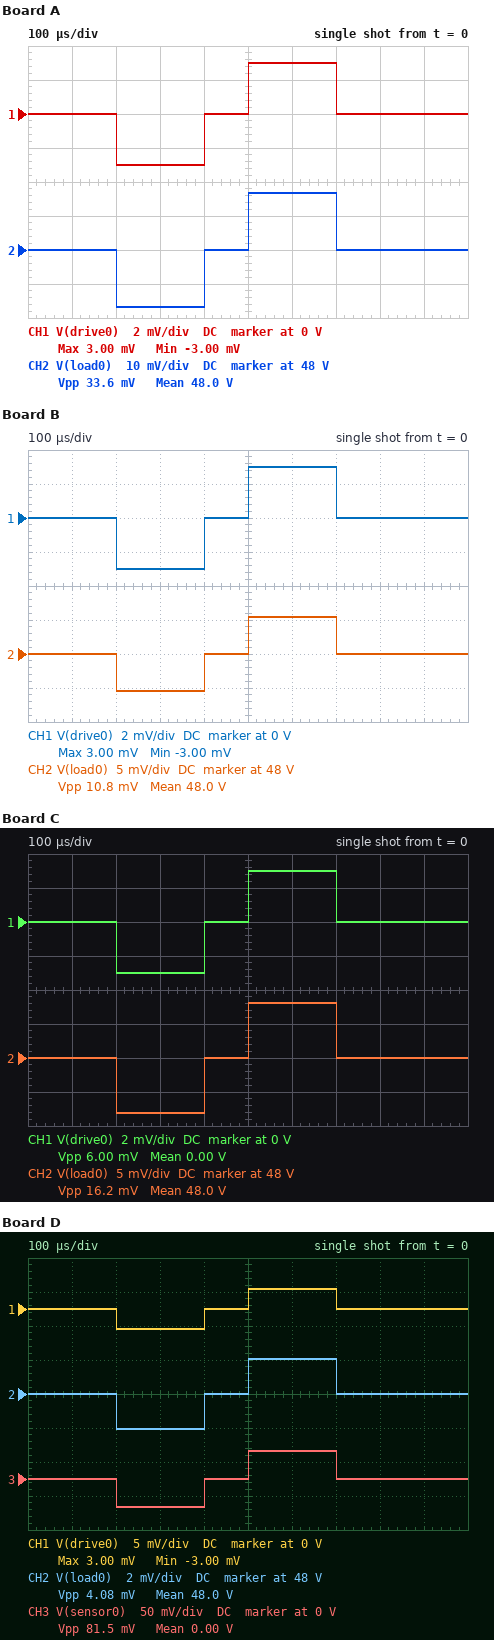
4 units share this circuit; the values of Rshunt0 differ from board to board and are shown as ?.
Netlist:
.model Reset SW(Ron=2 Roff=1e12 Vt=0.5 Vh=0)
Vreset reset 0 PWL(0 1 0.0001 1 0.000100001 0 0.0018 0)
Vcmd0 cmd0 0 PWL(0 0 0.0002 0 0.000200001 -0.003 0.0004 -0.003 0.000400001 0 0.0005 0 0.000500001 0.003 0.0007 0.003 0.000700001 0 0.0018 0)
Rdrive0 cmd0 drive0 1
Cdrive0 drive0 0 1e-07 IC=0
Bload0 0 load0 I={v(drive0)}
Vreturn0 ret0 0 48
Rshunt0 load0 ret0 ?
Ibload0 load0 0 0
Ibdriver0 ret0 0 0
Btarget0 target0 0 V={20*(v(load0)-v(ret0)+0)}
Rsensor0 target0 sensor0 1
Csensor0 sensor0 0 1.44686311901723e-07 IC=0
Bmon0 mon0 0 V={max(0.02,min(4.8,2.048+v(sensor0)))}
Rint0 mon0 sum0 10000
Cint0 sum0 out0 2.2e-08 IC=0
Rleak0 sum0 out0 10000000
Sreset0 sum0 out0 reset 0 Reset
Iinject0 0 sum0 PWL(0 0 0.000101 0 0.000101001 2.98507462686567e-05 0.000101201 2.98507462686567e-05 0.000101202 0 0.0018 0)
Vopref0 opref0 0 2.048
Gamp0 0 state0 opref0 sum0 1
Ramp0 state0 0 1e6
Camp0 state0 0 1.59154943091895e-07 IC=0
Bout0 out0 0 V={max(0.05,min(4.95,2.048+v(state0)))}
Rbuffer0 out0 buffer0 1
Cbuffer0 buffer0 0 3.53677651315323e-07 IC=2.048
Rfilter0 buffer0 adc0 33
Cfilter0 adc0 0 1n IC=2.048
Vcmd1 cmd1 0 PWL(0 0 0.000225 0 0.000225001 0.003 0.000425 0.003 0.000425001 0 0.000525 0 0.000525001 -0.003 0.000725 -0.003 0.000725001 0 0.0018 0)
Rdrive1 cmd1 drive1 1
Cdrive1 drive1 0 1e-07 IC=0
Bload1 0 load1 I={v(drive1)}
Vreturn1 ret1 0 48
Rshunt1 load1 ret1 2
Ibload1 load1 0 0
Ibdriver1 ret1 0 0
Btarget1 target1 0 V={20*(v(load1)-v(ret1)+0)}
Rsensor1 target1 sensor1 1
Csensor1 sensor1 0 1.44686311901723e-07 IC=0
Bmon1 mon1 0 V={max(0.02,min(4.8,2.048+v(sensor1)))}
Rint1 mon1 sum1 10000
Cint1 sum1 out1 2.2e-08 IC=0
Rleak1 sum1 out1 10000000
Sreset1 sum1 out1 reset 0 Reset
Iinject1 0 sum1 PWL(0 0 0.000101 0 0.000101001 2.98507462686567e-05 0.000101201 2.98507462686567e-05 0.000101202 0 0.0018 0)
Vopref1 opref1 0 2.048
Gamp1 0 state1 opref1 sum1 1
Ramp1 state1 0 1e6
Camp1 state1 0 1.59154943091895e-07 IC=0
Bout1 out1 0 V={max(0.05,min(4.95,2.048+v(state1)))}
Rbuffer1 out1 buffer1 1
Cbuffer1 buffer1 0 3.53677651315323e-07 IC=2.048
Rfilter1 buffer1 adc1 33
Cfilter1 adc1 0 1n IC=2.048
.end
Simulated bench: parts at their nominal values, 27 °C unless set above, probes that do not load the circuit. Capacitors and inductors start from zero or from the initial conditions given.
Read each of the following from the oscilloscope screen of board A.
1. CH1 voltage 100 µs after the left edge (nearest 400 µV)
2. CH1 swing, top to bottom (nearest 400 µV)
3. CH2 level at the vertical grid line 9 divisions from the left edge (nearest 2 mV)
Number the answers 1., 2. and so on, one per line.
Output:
1. 0 V
2. 6.0 mV
3. 48.000 V
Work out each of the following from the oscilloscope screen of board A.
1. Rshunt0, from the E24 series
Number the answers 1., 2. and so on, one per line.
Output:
1. 5.6 Ω
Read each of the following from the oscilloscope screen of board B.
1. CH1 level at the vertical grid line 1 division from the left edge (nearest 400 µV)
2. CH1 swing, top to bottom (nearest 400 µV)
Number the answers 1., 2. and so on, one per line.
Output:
1. 0 V
2. 6.0 mV
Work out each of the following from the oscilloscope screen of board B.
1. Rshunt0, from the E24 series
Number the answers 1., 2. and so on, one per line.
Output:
1. 1.8 Ω
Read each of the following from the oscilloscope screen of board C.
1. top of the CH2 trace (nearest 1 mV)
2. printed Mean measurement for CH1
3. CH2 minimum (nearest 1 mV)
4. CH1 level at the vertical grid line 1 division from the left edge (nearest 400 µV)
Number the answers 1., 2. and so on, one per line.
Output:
1. 48.008 V
2. 0.00 V
3. 47.992 V
4. 0 V
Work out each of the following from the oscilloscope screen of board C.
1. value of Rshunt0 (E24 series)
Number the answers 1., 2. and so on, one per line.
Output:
1. 2.7 Ω
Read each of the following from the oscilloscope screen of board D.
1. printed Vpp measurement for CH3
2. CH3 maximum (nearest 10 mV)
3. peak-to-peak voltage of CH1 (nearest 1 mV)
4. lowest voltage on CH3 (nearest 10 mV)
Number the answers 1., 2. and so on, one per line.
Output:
1. 81.5 mV
2. 40 mV
3. 6 mV
4. -40 mV
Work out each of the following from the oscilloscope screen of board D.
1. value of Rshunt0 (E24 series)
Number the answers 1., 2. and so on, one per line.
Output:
1. 0.68 Ω
